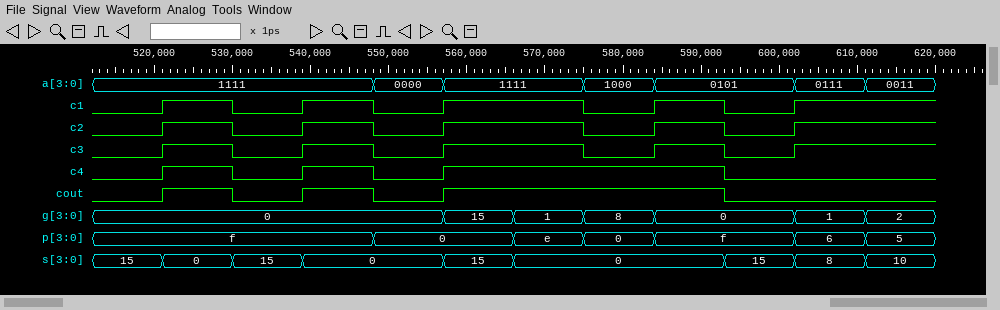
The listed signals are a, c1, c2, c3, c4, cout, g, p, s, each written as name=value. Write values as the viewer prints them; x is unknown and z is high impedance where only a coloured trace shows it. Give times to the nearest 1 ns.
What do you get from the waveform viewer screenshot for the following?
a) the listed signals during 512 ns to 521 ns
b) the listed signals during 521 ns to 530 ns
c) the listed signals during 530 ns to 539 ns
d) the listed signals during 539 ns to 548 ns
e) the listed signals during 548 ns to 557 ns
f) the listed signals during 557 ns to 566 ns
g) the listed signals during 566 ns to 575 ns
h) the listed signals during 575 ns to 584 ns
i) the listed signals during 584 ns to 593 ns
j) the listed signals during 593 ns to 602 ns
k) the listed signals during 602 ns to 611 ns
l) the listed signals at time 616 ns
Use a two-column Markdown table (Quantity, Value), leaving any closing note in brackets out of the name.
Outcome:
| Quantity | Value |
|---|---|
| the listed signals during 512 ns to 521 ns | a=1111, c1=0, c2=0, c3=0, c4=0, cout=0, g=0, p=f, s=15 |
| the listed signals during 521 ns to 530 ns | a=1111, c1=1, c2=1, c3=1, c4=1, cout=1, g=0, p=f, s=0 |
| the listed signals during 530 ns to 539 ns | a=1111, c1=0, c2=0, c3=0, c4=0, cout=0, g=0, p=f, s=15 |
| the listed signals during 539 ns to 548 ns | a=1111, c1=1, c2=1, c3=1, c4=1, cout=1, g=0, p=f, s=0 |
| the listed signals during 548 ns to 557 ns | a=0000, c1=0, c2=0, c3=0, c4=0, cout=0, g=0, p=0, s=0 |
| the listed signals during 557 ns to 566 ns | a=1111, c1=1, c2=1, c3=1, c4=1, cout=1, g=15, p=0, s=15 |
| the listed signals during 566 ns to 575 ns | a=1111, c1=1, c2=1, c3=1, c4=1, cout=1, g=1, p=e, s=0 |
| the listed signals during 575 ns to 584 ns | a=1000, c1=0, c2=0, c3=0, c4=1, cout=1, g=8, p=0, s=0 |
| the listed signals during 584 ns to 593 ns | a=0101, c1=1, c2=1, c3=1, c4=1, cout=1, g=0, p=f, s=0 |
| the listed signals during 593 ns to 602 ns | a=0101, c1=0, c2=0, c3=0, c4=0, cout=0, g=0, p=f, s=15 |
| the listed signals during 602 ns to 611 ns | a=0111, c1=1, c2=1, c3=1, c4=0, cout=0, g=1, p=6, s=8 |
| the listed signals at time 616 ns | a=0011, c1=1, c2=1, c3=1, c4=0, cout=0, g=2, p=5, s=10 |
